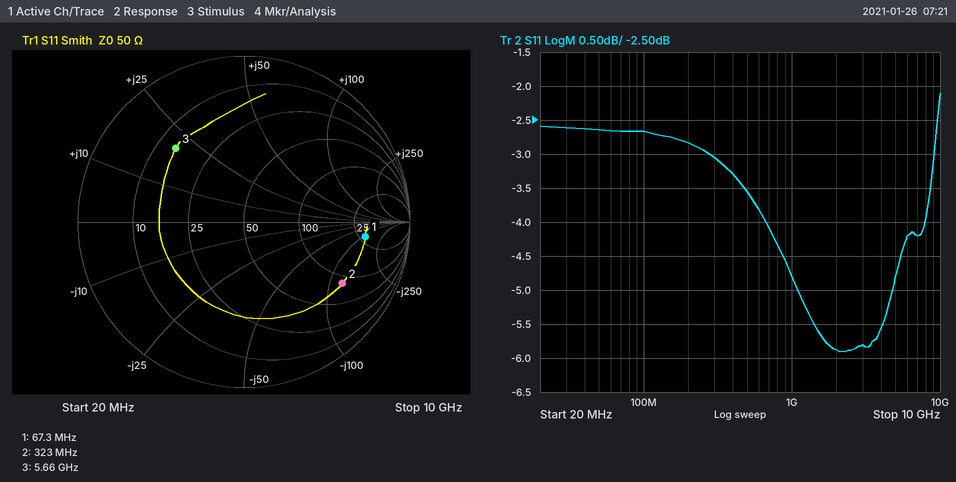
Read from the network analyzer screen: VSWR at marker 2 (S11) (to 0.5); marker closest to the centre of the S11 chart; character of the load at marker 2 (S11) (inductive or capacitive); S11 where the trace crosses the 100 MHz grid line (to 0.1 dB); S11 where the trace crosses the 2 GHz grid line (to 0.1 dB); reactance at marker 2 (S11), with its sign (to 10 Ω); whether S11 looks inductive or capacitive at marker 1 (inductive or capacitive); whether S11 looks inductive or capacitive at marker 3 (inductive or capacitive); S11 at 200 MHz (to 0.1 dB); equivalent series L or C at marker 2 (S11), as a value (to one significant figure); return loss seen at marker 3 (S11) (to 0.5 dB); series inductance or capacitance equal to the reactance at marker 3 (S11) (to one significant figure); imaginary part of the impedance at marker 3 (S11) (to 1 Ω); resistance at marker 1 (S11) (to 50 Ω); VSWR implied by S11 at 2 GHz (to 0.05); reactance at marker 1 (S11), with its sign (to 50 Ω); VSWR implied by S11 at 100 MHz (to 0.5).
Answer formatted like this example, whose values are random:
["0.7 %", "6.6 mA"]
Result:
["5.5", "marker 3", "capacitive", "-2.7 dB", "-5.9 dB", "-120 Ω", "capacitive", "inductive", "-2.8 dB", "4 pF", "4.5 dB", "600 pH", "+20 Ω", "300 Ω", "3.05", "-100 Ω", "6.5"]
